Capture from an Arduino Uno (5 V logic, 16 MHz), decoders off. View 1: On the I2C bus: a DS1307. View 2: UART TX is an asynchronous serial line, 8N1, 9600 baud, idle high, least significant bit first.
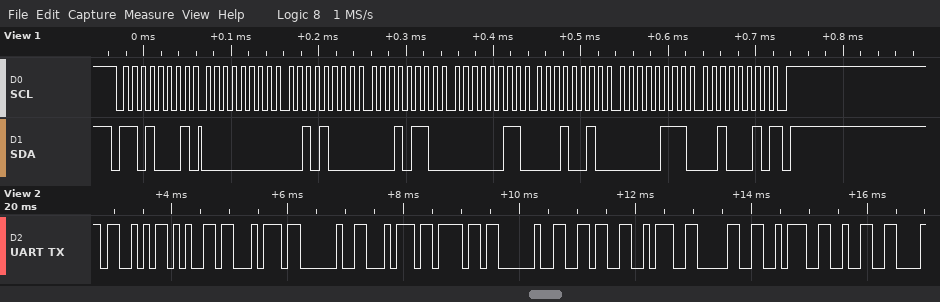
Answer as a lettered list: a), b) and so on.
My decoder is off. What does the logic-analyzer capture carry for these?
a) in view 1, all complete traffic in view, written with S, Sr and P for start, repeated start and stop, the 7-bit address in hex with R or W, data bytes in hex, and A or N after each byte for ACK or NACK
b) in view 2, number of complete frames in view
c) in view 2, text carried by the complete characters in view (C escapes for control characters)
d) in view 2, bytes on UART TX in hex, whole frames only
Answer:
a) S 68R A 00 A 28 A 16 A 03 A 12 A 07 A 22 N P
b) 12
c) "Set to 6:0:2"
d) 53 65 74 20 74 6F 20 36 3A 30 3A 32
